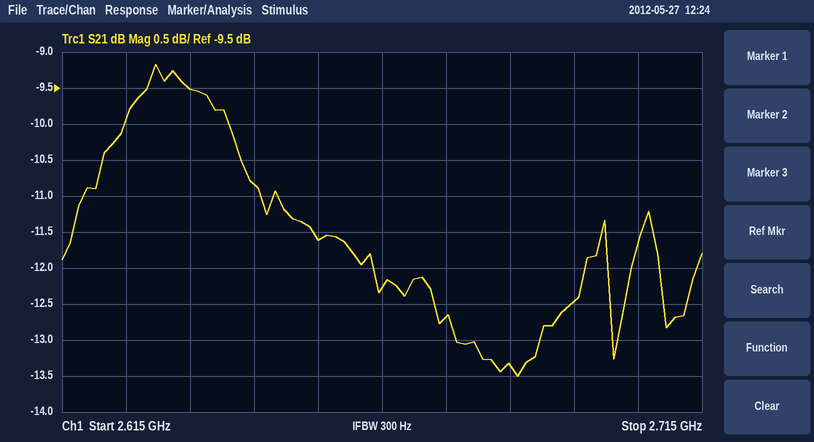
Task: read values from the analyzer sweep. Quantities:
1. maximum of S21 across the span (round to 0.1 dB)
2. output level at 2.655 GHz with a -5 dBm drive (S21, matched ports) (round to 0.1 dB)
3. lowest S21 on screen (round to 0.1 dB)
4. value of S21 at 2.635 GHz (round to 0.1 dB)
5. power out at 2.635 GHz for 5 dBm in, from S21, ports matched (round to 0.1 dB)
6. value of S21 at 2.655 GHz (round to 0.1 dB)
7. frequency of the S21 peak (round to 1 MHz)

-9.2 dB
-16.6 dBm
-13.5 dB
-9.5 dB
-4.5 dBm
-11.6 dB
2.630 GHz
